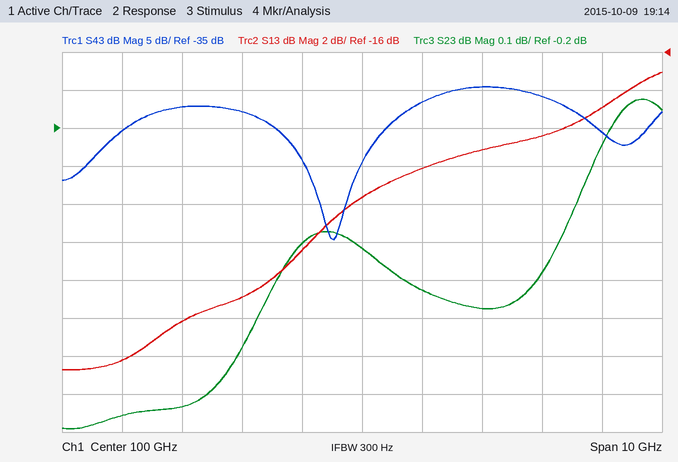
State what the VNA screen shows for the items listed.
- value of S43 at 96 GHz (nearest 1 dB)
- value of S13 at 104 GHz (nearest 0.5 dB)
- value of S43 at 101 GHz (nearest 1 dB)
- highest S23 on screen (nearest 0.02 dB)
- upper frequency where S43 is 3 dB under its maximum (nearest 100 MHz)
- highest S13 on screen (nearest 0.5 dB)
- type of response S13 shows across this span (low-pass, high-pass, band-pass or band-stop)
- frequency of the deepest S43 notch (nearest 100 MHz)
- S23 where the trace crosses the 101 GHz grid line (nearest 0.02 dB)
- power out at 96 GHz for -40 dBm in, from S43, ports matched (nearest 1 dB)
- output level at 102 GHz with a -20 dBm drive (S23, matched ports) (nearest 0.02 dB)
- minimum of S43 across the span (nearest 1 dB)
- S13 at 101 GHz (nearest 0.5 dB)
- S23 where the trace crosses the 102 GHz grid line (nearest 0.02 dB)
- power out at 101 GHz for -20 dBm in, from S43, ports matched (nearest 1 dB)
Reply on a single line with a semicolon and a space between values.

-35 dB; -19.0 dB; -32 dB; -0.12 dB; 103.5 GHz; -17.0 dB; high-pass; 99.5 GHz; -0.62 dB; -75 dBm; -20.68 dBm; -50 dB; -22.0 dB; -0.68 dB; -52 dBm
